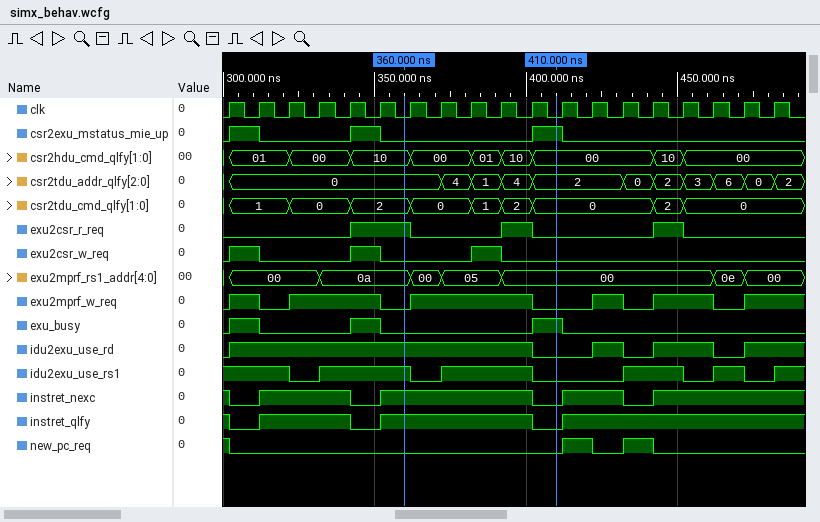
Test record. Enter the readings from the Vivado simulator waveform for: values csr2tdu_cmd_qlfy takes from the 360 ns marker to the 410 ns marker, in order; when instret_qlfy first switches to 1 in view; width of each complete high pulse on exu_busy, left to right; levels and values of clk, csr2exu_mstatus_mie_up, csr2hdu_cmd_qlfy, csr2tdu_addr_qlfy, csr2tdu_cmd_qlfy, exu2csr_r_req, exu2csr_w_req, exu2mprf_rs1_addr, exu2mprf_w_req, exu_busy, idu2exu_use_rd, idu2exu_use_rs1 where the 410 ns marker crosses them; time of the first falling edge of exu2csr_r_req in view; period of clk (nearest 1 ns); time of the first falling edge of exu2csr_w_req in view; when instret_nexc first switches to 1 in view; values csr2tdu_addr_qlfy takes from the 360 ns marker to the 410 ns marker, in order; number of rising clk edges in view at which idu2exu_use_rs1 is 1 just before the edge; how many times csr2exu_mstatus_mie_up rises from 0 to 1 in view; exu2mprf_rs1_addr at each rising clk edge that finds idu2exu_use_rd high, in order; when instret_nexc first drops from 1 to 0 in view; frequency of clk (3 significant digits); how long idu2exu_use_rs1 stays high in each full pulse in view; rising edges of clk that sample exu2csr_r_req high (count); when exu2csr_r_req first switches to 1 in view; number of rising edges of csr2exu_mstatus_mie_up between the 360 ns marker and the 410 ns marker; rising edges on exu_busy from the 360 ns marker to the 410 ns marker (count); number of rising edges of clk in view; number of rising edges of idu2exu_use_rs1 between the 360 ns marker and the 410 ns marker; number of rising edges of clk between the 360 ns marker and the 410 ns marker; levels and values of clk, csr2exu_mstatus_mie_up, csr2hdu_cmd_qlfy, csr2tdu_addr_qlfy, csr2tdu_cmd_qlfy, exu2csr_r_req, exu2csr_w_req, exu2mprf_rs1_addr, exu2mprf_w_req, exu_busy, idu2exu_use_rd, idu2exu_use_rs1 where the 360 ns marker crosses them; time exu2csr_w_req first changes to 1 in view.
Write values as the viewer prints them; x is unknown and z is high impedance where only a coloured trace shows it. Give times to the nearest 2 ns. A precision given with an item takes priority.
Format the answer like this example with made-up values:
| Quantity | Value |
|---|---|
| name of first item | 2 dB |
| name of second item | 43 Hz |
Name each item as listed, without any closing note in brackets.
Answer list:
| Quantity | Value |
|---|---|
| values csr2tdu_cmd_qlfy takes from the 360 ns marker to the 410 ns marker, in order | 2, 0, 1, 2, 0 |
| when instret_qlfy first switches to 1 in view | 312 ns |
| width of each complete high pulse on exu_busy, left to right | 10 ns, 10 ns, 10 ns |
| levels and values of clk, csr2exu_mstatus_mie_up, csr2hdu_cmd_qlfy, csr2tdu_addr_qlfy, csr2tdu_cmd_qlfy, exu2csr_r_req, exu2csr_w_req, exu2mprf_rs1_addr, exu2mprf_w_req, exu_busy, idu2exu_use_rd, idu2exu_use_rs1 where the 410 ns marker crosses them | clk=0, csr2exu_mstatus_mie_up=1, csr2hdu_cmd_qlfy=00, csr2tdu_addr_qlfy=2, csr2tdu_cmd_qlfy=0, exu2csr_r_req=0, exu2csr_w_req=0, exu2mprf_rs1_addr=00, exu2mprf_w_req=0, exu_busy=1, idu2exu_use_rd=0, idu2exu_use_rs1=0 |
| time of the first falling edge of exu2csr_r_req in view | 362 ns |
| period of clk | 10 ns |
| time of the first falling edge of exu2csr_w_req in view | 312 ns |
| when instret_nexc first switches to 1 in view | 312 ns |
| values csr2tdu_addr_qlfy takes from the 360 ns marker to the 410 ns marker, in order | 0, 4, 1, 4, 2 |
| number of rising clk edges in view at which idu2exu_use_rs1 is 1 just before the edge | 12 |
| how many times csr2exu_mstatus_mie_up rises from 0 to 1 in view | 3 |
| exu2mprf_rs1_addr at each rising clk edge that finds idu2exu_use_rd high, in order | 00, 00, 00, 0a, 0a, 0a, 00, 05, 05, 00, 00, 00, 00, 00 |
| when instret_nexc first drops from 1 to 0 in view | 302 ns |
| frequency of clk | 100 MHz |
| how long idu2exu_use_rs1 stays high in each full pulse in view | 30 ns, 30 ns, 20 ns, 10 ns |
| rising edges of clk that sample exu2csr_r_req high | 4 |
| when exu2csr_r_req first switches to 1 in view | 342 ns |
| number of rising edges of csr2exu_mstatus_mie_up between the 360 ns marker and the 410 ns marker | 1 |
| rising edges on exu_busy from the 360 ns marker to the 410 ns marker | 1 |
| number of rising edges of clk in view | 19 |
| number of rising edges of idu2exu_use_rs1 between the 360 ns marker and the 410 ns marker | 1 |
| number of rising edges of clk between the 360 ns marker and the 410 ns marker | 5 |
| levels and values of clk, csr2exu_mstatus_mie_up, csr2hdu_cmd_qlfy, csr2tdu_addr_qlfy, csr2tdu_cmd_qlfy, exu2csr_r_req, exu2csr_w_req, exu2mprf_rs1_addr, exu2mprf_w_req, exu_busy, idu2exu_use_rd, idu2exu_use_rs1 where the 360 ns marker crosses them | clk=0, csr2exu_mstatus_mie_up=0, csr2hdu_cmd_qlfy=10, csr2tdu_addr_qlfy=0, csr2tdu_cmd_qlfy=2, exu2csr_r_req=1, exu2csr_w_req=0, exu2mprf_rs1_addr=0a, exu2mprf_w_req=0, exu_busy=0, idu2exu_use_rd=1, idu2exu_use_rs1=1 |
| time exu2csr_w_req first changes to 1 in view | 302 ns |
